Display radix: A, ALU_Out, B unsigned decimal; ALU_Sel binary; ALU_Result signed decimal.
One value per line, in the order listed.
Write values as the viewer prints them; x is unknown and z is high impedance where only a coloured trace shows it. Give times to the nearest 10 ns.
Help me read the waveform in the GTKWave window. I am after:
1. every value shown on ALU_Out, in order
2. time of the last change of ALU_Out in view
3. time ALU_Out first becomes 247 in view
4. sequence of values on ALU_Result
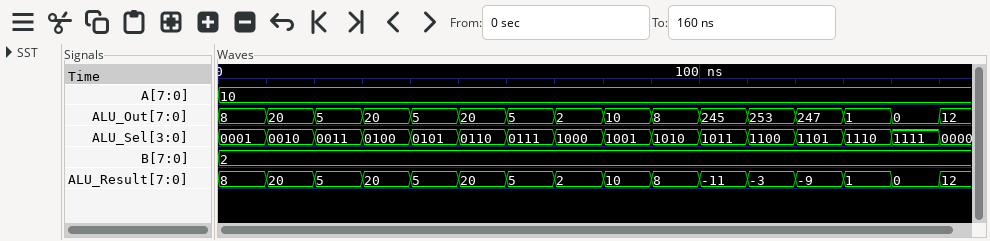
8, 20, 5, 20, 5, 20, 5, 2, 10, 8, 245, 253, 247, 1, 0, 12
150 ns
120 ns
8, 20, 5, 20, 5, 20, 5, 2, 10, 8, -11, -3, -9, 1, 0, 12
